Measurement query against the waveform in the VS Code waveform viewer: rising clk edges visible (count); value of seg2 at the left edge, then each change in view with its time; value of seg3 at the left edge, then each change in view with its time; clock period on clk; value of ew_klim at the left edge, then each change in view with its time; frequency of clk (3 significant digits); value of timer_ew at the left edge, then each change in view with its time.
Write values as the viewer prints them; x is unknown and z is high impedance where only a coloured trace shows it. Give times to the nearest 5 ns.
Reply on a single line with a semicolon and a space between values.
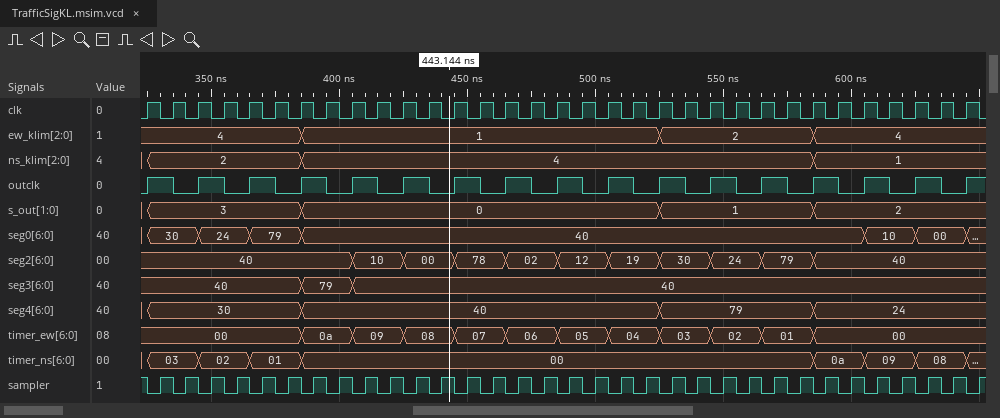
33; 40, 10 at 405 ns, 00 at 425 ns, 78 at 445 ns, 02 at 465 ns, 12 at 485 ns, 19 at 505 ns, 30 at 525 ns, 24 at 545 ns, 79 at 565 ns, 40 at 585 ns; 40, 79 at 385 ns, 40 at 405 ns; 10 ns; 4, 1 at 385 ns, 2 at 525 ns, 4 at 585 ns; 100 MHz; 00, 0a at 385 ns, 09 at 405 ns, 08 at 425 ns, 07 at 445 ns, 06 at 465 ns, 05 at 485 ns, 04 at 505 ns, 03 at 525 ns, 02 at 545 ns, 01 at 565 ns, 00 at 585 ns
